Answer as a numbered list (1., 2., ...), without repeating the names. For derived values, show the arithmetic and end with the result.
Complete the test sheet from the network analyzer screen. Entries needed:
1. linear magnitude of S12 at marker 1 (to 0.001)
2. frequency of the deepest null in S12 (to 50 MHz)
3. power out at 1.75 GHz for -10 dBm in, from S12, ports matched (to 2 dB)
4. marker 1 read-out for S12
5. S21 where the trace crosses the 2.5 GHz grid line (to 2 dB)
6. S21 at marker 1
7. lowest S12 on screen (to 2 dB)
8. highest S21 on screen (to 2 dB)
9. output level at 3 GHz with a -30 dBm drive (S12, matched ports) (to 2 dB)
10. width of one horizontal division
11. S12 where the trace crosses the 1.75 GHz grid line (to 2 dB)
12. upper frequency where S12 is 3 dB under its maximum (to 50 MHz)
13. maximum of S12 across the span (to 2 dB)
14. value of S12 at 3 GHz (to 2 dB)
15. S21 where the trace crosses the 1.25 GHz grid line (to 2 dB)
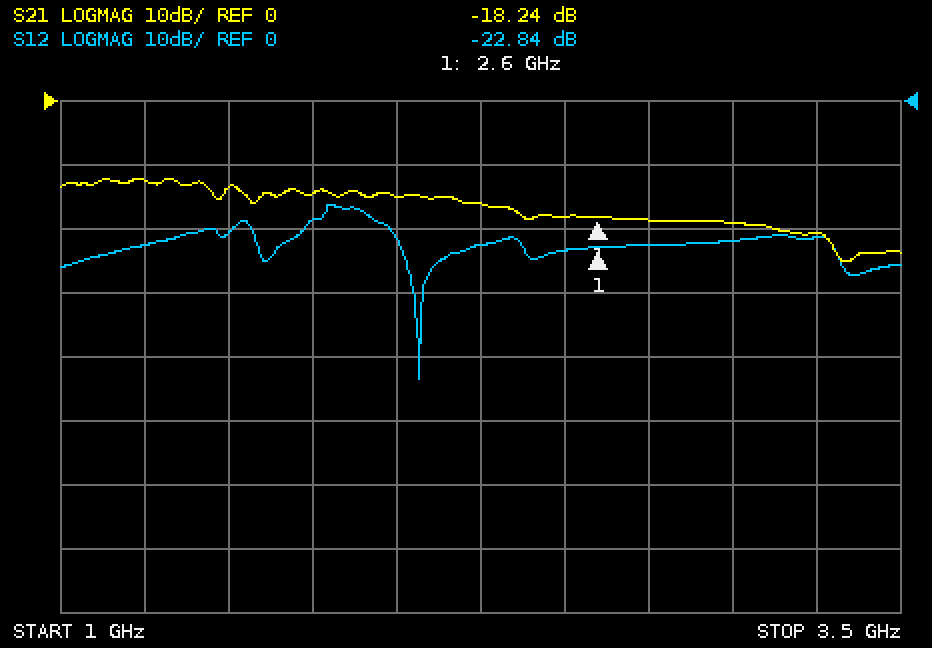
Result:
1. 10^(-22.84/20) ≈ 0.072
2. 2.05 GHz
3. -10 dBm + (-18 dB) = -28 dBm
4. -22.84 dB
5. -18 dB
6. -18.24 dB
7. -44 dB
8. -12 dB
9. -30 dBm + (-22 dB) = -52 dBm
10. 250 MHz
11. -18 dB
12. 1.95 GHz
13. -16 dB
14. -22 dB
15. -12 dB
